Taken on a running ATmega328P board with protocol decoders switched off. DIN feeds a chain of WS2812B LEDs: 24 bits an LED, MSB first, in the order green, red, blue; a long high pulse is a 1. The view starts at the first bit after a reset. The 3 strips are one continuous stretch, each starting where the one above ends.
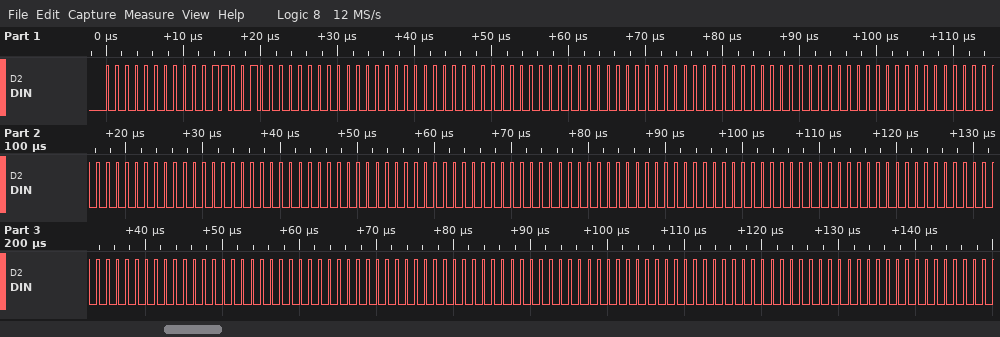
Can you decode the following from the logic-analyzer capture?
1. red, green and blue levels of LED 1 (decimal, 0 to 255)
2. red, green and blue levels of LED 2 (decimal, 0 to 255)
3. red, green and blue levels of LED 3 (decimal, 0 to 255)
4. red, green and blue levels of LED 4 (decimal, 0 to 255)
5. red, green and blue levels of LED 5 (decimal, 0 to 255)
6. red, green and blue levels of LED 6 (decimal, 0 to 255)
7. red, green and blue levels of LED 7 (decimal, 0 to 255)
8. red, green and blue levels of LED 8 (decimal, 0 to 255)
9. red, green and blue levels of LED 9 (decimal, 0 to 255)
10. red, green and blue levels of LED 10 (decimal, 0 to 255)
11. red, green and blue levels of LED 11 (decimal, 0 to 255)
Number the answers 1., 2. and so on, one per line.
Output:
1. 25, 0, 0
2. 0, 0, 0
3. 0, 0, 0
4. 0, 0, 0
5. 0, 0, 0
6. 0, 0, 0
7. 0, 0, 0
8. 0, 0, 0
9. 0, 0, 0
10. 0, 0, 0
11. 0, 0, 0
